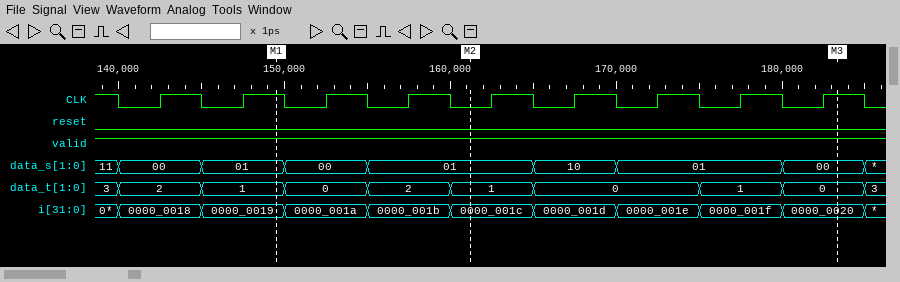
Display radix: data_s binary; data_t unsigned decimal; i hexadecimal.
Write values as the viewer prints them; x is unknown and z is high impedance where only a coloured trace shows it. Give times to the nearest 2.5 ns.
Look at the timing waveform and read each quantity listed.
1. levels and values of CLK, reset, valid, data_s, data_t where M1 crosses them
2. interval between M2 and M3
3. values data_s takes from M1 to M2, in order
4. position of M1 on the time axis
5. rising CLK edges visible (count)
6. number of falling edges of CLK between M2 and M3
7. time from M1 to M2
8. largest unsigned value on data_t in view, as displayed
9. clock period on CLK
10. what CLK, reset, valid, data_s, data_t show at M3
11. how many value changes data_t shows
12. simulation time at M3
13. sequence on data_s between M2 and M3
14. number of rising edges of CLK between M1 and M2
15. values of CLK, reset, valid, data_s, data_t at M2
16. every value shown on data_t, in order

CLK=1, reset=0, valid=1, data_s=01, data_t=1
22.5 ns
01, 00, 01
150 ns
9
4
12.5 ns
3
5 ns
CLK=1, reset=0, valid=1, data_s=00, data_t=0
9
182.5 ns
01, 10, 01, 00
2
CLK=0, reset=0, valid=1, data_s=01, data_t=1
3, 2, 1, 0, 2, 1, 0, 1, 0, 3
